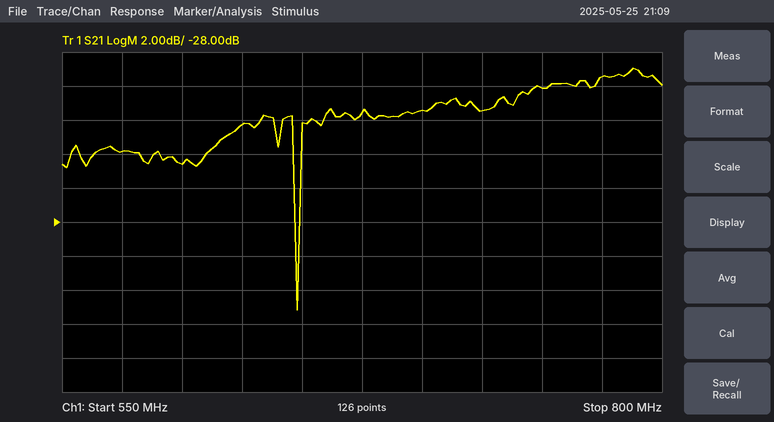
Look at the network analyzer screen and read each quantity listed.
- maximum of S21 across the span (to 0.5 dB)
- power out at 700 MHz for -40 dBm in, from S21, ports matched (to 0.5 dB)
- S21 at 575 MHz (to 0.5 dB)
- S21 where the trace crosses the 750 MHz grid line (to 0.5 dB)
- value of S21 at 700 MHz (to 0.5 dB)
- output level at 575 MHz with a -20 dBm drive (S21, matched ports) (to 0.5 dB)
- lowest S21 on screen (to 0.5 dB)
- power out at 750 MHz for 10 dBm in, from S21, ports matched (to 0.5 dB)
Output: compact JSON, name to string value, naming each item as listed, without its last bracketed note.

{"maximum of S21 across the span": "-19.0 dB", "power out at 700 MHz for -40 dBm in, from S21, ports matched": "-61.5 dBm", "S21 at 575 MHz": "-24.0 dB", "S21 where the trace crosses the 750 MHz grid line": "-20.0 dB", "value of S21 at 700 MHz": "-21.5 dB", "output level at 575 MHz with a -20 dBm drive (S21, matched ports)": "-44.0 dBm", "lowest S21 on screen": "-33.0 dB", "power out at 750 MHz for 10 dBm in, from S21, ports matched": "-10.0 dBm"}
